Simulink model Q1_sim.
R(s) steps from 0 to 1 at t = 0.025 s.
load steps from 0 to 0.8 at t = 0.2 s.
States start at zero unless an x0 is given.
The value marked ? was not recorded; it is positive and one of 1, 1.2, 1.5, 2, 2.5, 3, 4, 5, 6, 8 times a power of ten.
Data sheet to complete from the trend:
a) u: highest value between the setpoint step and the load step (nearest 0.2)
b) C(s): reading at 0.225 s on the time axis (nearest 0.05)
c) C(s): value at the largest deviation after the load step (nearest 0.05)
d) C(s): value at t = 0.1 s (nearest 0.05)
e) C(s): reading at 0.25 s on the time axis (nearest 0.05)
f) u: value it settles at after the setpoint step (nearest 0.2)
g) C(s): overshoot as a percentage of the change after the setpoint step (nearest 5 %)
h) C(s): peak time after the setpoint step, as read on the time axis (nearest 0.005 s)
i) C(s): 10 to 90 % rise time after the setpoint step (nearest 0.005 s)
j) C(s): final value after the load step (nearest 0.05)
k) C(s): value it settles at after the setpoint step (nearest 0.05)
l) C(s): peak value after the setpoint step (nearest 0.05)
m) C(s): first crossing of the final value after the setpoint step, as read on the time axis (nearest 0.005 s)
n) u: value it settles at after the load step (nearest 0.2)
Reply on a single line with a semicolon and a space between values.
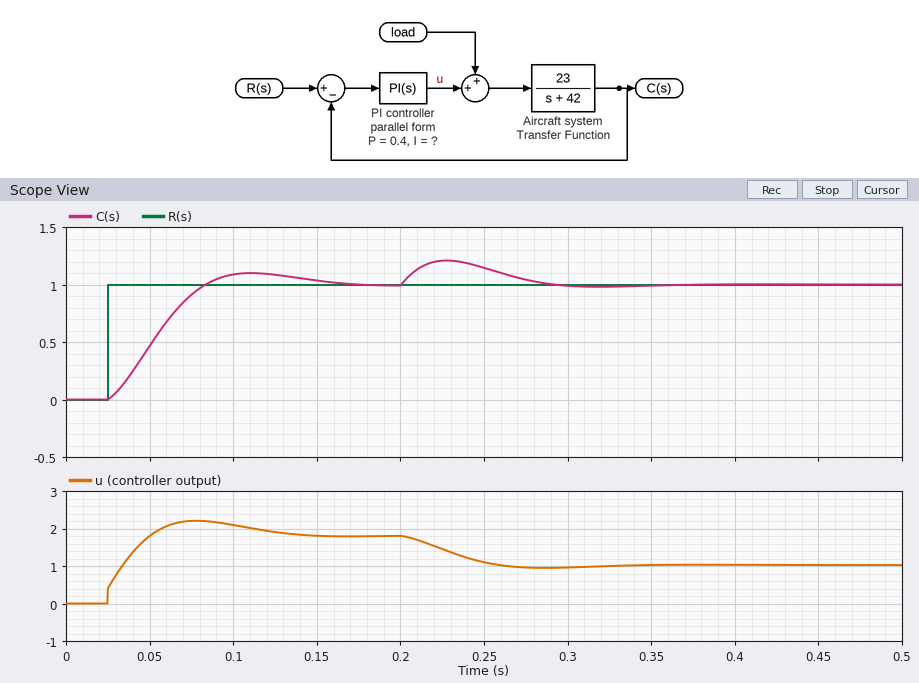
2.2; 1.20; 1.20; 1.10; 1.15; 1.8; 10 %; 0.110 s; 0.040 s; 1.00; 1.00; 1.10; 0.085 s; 1.0
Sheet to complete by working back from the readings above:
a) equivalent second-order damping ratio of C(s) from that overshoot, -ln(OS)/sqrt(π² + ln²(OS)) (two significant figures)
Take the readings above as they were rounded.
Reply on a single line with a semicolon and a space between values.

0.59
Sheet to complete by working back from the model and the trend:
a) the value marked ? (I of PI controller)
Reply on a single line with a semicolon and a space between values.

80
